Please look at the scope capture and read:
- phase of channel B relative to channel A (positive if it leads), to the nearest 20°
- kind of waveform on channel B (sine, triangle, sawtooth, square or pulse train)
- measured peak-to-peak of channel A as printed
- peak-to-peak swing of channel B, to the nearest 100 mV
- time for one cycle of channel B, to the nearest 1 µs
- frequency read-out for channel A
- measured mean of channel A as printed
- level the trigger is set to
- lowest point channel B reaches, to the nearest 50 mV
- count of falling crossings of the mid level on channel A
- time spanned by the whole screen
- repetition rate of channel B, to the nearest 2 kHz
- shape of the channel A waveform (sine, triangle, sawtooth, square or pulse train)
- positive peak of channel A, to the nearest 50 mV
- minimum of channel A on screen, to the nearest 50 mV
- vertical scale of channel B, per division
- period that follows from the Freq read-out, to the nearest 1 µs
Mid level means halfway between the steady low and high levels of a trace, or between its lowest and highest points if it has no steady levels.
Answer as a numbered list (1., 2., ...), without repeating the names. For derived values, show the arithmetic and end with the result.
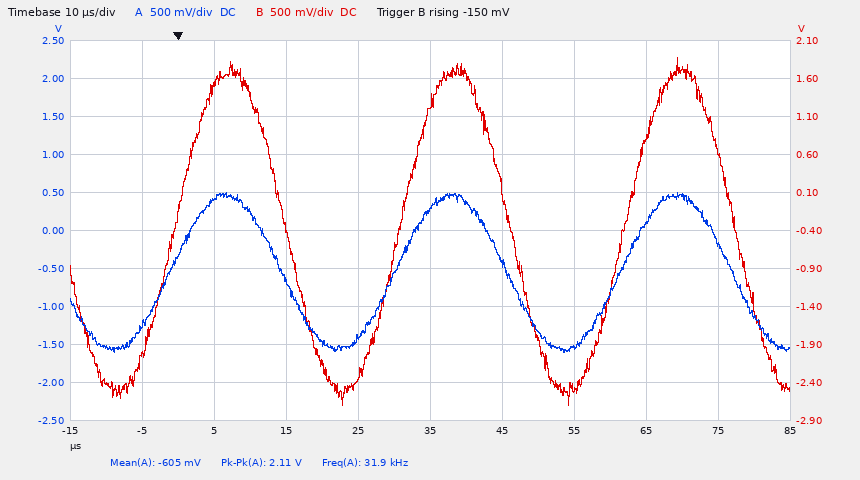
1. 0°
2. sine
3. 2.11 V
4. 4.60 V
5. 31 µs
6. 31.9 kHz
7. -605 mV
8. -150 mV
9. -2.70 V
10. 3
11. 100 µs
12. 1 / 31 µs ≈ 32 kHz
13. sine
14. 500 mV
15. -1.60 V
16. 500 mV
17. 1 / 31.9 kHz ≈ 31 µs
